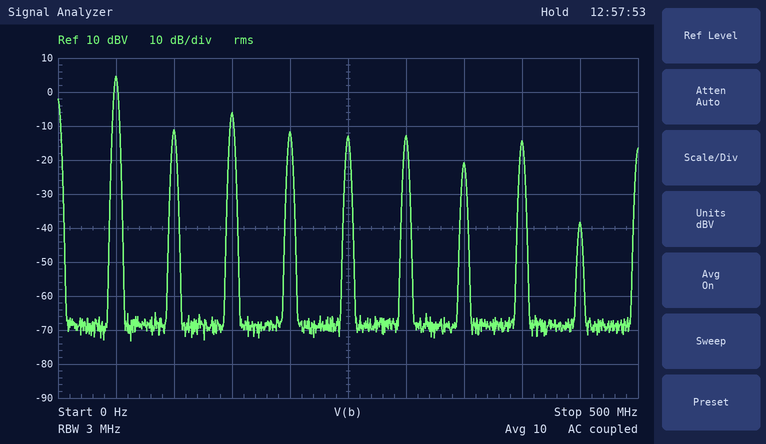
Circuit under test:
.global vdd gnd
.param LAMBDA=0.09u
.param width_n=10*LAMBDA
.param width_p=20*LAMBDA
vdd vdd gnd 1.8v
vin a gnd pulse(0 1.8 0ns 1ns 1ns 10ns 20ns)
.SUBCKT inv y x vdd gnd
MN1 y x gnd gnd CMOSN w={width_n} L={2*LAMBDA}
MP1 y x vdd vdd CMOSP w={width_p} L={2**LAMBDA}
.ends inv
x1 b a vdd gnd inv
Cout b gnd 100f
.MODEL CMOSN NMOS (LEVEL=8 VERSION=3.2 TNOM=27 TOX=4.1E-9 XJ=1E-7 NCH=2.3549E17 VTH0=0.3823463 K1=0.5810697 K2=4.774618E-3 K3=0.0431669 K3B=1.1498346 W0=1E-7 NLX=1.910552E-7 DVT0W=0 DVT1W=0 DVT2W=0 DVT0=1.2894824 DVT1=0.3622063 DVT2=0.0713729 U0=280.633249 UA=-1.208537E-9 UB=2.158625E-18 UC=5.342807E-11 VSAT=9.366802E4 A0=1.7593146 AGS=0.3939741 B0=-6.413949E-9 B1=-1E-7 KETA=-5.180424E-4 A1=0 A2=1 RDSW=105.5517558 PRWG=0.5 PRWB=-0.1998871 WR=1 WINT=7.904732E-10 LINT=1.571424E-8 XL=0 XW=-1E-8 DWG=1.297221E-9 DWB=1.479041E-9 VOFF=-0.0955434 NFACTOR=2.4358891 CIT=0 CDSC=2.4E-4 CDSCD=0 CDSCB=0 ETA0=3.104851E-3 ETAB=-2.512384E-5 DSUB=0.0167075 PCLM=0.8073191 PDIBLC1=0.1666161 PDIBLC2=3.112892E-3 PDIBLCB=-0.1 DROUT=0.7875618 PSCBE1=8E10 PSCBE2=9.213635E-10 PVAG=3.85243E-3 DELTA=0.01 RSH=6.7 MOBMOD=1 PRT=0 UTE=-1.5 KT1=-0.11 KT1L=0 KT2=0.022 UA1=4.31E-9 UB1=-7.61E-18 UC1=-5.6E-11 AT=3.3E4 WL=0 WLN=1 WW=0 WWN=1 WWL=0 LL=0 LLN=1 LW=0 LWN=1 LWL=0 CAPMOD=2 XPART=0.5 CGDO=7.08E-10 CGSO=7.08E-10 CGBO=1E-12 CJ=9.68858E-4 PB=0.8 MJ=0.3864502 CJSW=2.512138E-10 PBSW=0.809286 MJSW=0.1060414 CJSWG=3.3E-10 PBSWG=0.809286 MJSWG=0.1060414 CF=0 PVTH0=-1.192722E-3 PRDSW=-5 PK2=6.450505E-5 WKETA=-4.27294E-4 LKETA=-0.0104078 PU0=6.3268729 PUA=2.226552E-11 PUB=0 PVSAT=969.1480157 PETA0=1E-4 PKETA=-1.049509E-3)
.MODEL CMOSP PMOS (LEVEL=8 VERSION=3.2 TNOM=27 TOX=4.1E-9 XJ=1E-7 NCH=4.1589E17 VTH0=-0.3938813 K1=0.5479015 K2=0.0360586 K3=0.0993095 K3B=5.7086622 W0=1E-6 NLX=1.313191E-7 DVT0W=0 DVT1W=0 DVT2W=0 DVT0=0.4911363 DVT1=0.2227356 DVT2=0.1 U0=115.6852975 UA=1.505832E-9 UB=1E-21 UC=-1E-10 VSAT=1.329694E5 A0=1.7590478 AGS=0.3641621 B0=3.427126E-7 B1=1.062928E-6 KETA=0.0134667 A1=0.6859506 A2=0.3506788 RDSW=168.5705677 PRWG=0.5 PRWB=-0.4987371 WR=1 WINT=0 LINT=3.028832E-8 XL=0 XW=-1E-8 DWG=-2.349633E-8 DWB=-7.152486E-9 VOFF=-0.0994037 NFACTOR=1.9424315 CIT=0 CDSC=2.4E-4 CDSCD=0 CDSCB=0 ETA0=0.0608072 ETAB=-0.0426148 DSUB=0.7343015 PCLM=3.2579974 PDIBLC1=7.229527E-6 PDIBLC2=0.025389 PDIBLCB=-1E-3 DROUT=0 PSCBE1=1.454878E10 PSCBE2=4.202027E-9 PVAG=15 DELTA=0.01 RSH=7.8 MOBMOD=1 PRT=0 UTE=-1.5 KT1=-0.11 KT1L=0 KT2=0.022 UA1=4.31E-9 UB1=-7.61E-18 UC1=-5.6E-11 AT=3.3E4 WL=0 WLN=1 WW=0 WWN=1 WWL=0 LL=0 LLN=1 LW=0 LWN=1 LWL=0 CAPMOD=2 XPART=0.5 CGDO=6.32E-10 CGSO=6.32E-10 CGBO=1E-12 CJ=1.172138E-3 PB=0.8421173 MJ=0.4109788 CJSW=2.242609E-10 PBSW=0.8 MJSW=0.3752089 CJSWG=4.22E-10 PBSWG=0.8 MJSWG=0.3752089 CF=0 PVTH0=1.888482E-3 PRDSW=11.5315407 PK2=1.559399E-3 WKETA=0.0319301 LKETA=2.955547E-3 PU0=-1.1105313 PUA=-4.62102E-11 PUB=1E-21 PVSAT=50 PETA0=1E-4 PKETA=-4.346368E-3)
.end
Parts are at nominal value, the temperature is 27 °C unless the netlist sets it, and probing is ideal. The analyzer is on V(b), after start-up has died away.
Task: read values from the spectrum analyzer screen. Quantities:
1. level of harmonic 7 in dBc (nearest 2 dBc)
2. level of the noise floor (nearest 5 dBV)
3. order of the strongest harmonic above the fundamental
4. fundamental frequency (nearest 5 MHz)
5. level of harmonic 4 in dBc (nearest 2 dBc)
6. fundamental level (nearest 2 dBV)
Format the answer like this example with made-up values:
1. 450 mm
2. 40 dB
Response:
1. -26 dBc
2. -70 dBV
3. 3
4. 50 MHz
5. -16 dBc
6. 4 dBV
